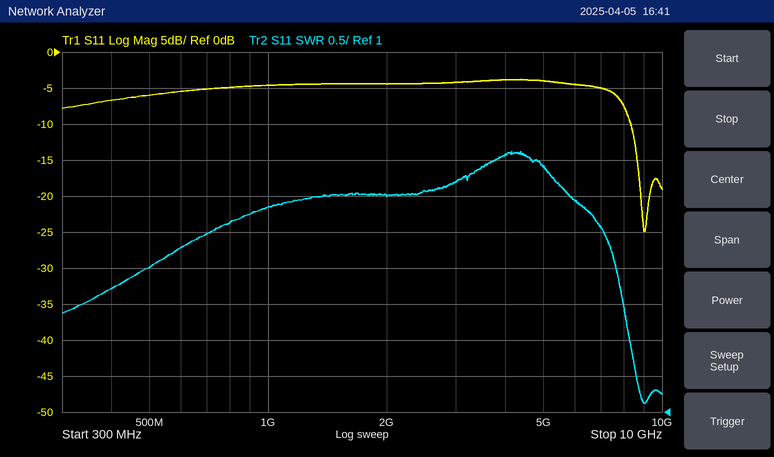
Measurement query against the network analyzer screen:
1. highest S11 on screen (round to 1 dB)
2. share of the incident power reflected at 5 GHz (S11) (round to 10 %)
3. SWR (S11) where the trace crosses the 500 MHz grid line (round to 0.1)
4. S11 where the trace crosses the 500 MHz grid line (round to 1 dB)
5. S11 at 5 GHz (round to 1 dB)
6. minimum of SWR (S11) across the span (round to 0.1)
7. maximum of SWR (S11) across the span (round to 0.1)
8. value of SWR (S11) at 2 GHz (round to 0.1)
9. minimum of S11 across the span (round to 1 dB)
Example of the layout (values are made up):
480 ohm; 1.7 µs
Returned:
-4 dB; 40 %; 3.0; -6 dB; -4 dB; 1.1; 4.6; 4.0; -25 dB
